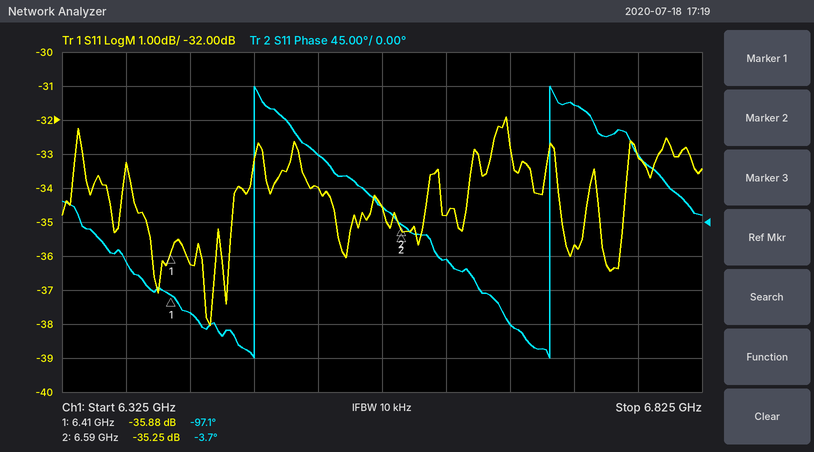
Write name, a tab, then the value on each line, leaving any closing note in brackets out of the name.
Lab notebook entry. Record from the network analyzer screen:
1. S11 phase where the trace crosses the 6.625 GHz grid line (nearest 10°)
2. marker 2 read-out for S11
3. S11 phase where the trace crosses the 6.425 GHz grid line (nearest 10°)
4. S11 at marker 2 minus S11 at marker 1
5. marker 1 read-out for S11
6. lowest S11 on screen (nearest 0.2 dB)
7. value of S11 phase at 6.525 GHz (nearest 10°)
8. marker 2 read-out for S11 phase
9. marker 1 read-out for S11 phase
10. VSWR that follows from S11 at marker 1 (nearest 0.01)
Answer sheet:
S11 phase where the trace crosses the 6.625 GHz grid line	-50°
marker 2 read-out for S11	-35.25 dB
S11 phase where the trace crosses the 6.425 GHz grid line	-120°
S11 at marker 2 minus S11 at marker 1	0.63 dB
marker 1 read-out for S11	-35.88 dB
lowest S11 on screen	-38.0 dB
value of S11 phase at 6.525 GHz	90°
marker 2 read-out for S11 phase	-3.7°
marker 1 read-out for S11 phase	-97.1°
VSWR that follows from S11 at marker 1	1.03
